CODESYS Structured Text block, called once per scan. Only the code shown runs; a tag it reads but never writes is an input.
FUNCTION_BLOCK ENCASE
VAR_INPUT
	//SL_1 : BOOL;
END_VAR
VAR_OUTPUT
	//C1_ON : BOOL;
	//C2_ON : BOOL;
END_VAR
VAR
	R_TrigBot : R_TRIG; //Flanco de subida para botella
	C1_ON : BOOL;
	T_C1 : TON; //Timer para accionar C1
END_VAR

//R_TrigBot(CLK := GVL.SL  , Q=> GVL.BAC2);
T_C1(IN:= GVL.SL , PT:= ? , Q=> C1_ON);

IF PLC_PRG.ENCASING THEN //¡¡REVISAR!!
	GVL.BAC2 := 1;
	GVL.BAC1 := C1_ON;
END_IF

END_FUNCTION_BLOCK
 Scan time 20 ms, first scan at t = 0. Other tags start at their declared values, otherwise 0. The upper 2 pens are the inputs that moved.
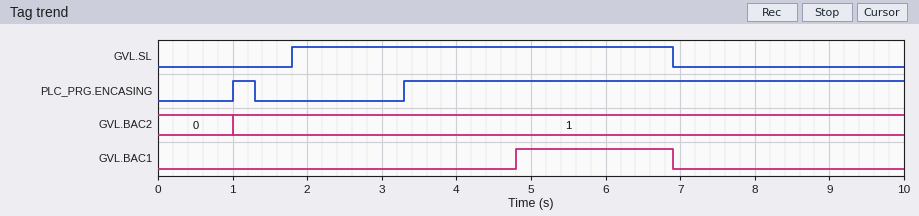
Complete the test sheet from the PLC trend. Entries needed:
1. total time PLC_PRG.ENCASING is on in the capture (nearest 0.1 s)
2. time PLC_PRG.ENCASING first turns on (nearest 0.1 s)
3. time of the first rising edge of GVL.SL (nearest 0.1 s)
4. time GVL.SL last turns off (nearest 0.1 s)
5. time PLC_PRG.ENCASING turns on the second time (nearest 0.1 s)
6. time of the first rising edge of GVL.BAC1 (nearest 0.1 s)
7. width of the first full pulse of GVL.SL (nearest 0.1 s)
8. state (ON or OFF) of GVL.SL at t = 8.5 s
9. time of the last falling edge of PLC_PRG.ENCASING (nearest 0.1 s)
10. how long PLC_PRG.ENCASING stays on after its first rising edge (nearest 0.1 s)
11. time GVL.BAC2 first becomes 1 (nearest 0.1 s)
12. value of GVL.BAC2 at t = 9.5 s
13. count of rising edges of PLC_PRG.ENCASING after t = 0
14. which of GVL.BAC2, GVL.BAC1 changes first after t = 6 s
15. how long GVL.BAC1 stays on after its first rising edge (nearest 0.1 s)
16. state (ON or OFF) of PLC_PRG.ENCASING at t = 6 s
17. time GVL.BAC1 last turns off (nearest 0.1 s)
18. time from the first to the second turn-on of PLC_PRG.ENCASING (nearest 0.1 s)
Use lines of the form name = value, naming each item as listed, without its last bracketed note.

total time PLC_PRG.ENCASING is on in the capture = 7.0 s
time PLC_PRG.ENCASING first turns on = 1.0 s
time of the first rising edge of GVL.SL = 1.8 s
time GVL.SL last turns off = 6.9 s
time PLC_PRG.ENCASING turns on the second time = 3.3 s
time of the first rising edge of GVL.BAC1 = 4.8 s
width of the first full pulse of GVL.SL = 5.1 s
state (ON or OFF) of GVL.SL at t = 8.5 s = OFF
time of the last falling edge of PLC_PRG.ENCASING = 1.3 s
how long PLC_PRG.ENCASING stays on after its first rising edge = 0.3 s
time GVL.BAC2 first becomes 1 = 1.0 s
value of GVL.BAC2 at t = 9.5 s = 1
count of rising edges of PLC_PRG.ENCASING after t = 0 = 2
which of GVL.BAC2, GVL.BAC1 changes first after t = 6 s = GVL.BAC1
how long GVL.BAC1 stays on after its first rising edge = 2.1 s
state (ON or OFF) of PLC_PRG.ENCASING at t = 6 s = ON
time GVL.BAC1 last turns off = 6.9 s
time from the first to the second turn-on of PLC_PRG.ENCASING = 2.3 s
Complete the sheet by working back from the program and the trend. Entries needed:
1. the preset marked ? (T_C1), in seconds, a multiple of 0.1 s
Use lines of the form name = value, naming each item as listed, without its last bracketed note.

the preset marked ? (T_C1), in seconds, a multiple of 0.1 s = 3.0 s
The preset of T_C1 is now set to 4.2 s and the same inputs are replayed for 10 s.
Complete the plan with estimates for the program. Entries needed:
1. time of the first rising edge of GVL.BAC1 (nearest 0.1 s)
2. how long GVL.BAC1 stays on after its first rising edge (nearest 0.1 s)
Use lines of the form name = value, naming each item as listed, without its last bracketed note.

time of the first rising edge of GVL.BAC1 = 6.0 s
how long GVL.BAC1 stays on after its first rising edge = 0.9 s
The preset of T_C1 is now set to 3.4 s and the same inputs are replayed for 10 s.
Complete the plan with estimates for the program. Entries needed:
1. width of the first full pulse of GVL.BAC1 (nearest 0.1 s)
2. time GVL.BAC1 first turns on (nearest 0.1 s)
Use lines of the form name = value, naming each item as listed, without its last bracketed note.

width of the first full pulse of GVL.BAC1 = 1.7 s
time GVL.BAC1 first turns on = 5.2 s
